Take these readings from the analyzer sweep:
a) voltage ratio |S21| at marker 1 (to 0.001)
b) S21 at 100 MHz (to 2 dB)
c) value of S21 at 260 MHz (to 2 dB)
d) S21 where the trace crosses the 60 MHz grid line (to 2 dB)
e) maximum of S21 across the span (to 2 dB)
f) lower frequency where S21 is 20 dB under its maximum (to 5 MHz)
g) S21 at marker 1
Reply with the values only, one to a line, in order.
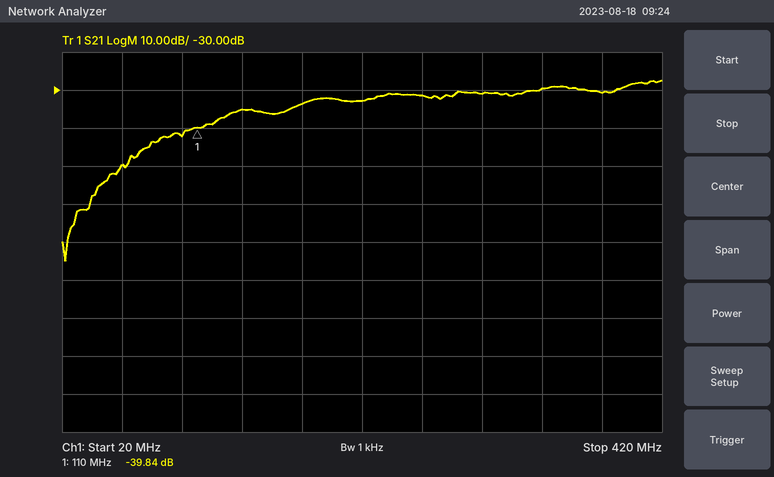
0.010
-42 dB
-32 dB
-50 dB
-28 dB
70 MHz
-39.84 dB
